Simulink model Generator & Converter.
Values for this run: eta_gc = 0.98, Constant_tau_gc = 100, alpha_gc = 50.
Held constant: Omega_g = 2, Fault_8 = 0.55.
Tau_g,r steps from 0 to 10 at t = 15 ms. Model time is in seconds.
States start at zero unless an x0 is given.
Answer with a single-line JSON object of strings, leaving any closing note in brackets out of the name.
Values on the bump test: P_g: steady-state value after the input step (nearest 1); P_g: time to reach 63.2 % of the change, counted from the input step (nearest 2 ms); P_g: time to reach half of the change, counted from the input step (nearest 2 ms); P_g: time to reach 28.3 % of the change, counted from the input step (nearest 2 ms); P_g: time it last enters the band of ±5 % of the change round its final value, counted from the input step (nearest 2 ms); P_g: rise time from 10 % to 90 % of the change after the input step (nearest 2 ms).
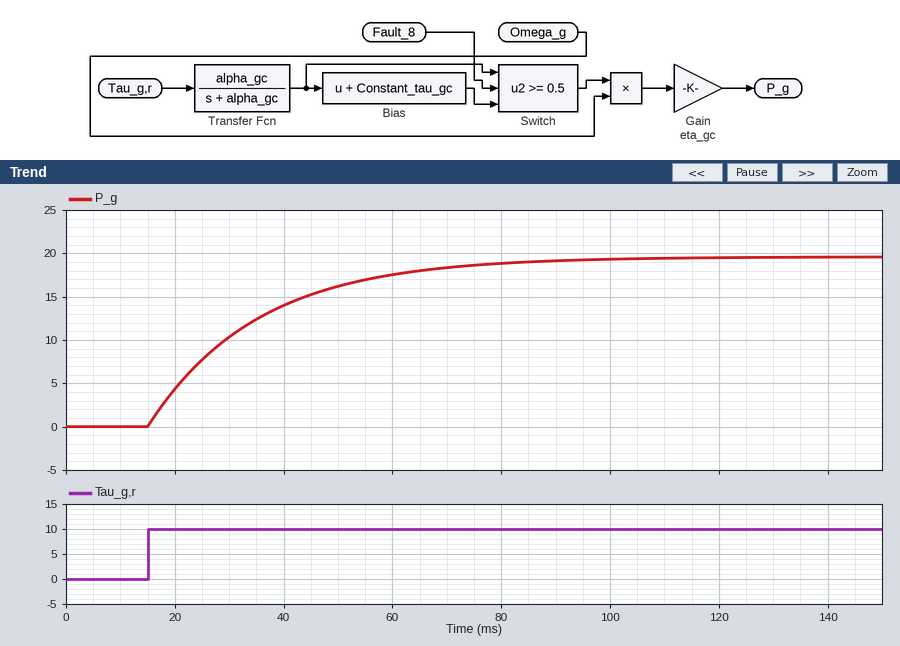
{"P_g: steady-state value after the input step": "20", "P_g: time to reach 63.2 % of the change, counted from the input step": "20 ms", "P_g: time to reach half of the change, counted from the input step": "14 ms", "P_g: time to reach 28.3 % of the change, counted from the input step": "6 ms", "P_g: time it last enters the band of ±5 % of the change round its final value, counted from the input step": "60 ms", "P_g: rise time from 10 % to 90 % of the change after the input step": "44 ms"}
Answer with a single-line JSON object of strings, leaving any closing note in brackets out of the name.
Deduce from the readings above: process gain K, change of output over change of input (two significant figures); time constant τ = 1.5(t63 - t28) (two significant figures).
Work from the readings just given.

{"process gain K, change of output over change of input": "2.0", "time constant τ = 1.5(t63 - t28)": "21 ms"}
